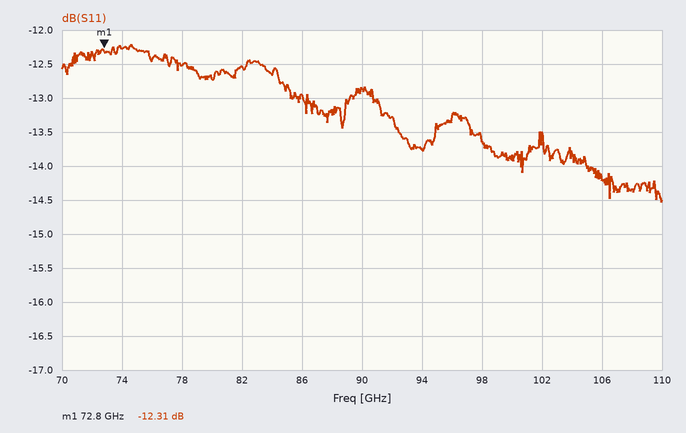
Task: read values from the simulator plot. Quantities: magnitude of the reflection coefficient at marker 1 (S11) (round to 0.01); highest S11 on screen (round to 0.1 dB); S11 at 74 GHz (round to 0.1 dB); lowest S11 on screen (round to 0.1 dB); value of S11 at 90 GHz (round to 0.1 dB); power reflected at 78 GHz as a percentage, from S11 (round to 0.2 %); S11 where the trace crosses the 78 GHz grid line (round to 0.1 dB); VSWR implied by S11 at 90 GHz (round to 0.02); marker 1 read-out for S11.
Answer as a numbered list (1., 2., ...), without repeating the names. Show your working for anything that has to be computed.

1. 10^(-12.31/20) ≈ 0.24
2. -12.2 dB
3. -12.3 dB
4. -14.5 dB
5. -12.9 dB
6. 10^(-12.5/10) ≈ 5.6 %
7. -12.5 dB
8. |Γ| = 10^(-12.9/20) = 0.2265; VSWR = (1 + 0.2265)/(1 − 0.2265) ≈ 1.59, so 1.58 to the nearest 0.02
9. -12.31 dB
